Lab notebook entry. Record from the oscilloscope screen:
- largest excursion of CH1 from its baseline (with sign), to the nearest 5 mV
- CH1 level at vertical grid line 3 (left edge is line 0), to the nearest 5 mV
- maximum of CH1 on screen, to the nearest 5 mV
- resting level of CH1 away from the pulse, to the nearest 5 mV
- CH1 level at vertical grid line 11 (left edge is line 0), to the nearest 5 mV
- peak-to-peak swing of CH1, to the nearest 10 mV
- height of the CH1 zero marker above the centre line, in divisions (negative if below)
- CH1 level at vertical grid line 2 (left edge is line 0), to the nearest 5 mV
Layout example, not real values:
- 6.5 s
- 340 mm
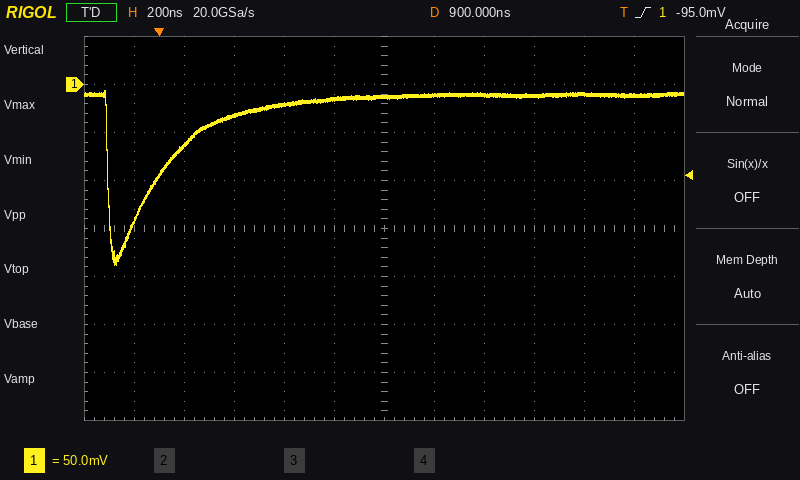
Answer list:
- -175 mV
- -30 mV
- -5 mV
- -10 mV
- -10 mV
- 180 mV
- +3.0 div
- -65 mV
